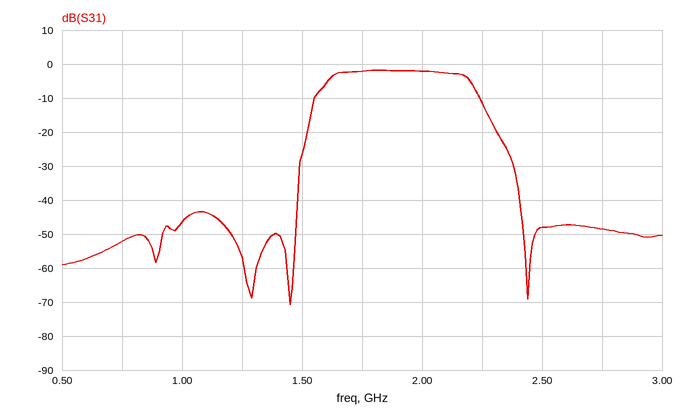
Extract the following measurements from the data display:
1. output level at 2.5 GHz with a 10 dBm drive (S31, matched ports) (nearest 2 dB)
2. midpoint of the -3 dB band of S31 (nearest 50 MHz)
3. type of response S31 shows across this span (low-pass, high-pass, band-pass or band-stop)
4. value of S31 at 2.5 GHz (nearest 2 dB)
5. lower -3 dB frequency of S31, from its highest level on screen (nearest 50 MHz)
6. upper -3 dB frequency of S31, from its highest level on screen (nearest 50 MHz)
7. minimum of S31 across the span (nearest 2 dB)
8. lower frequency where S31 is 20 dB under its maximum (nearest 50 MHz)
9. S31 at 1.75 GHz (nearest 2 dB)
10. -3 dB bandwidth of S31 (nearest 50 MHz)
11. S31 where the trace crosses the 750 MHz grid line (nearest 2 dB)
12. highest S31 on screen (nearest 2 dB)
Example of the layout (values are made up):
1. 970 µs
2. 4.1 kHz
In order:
1. -38 dBm
2. 1.90 GHz
3. band-pass
4. -48 dB
5. 1.60 GHz
6. 2.20 GHz
7. -70 dB
8. 1.50 GHz
9. -2 dB
10. 600 MHz
11. -52 dB
12. -2 dB
